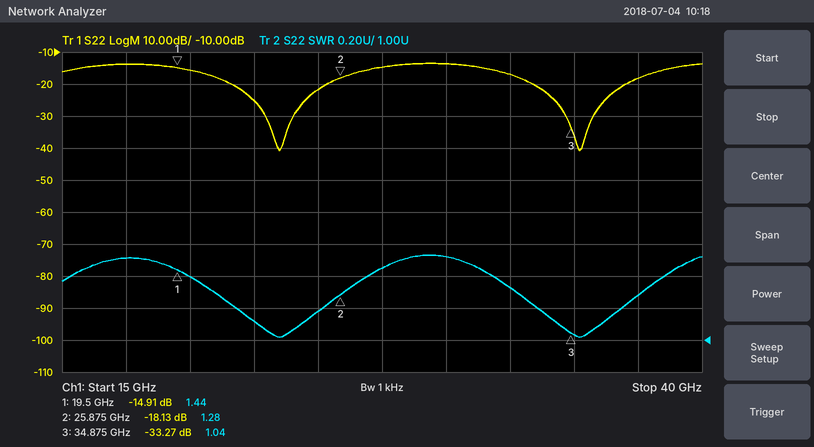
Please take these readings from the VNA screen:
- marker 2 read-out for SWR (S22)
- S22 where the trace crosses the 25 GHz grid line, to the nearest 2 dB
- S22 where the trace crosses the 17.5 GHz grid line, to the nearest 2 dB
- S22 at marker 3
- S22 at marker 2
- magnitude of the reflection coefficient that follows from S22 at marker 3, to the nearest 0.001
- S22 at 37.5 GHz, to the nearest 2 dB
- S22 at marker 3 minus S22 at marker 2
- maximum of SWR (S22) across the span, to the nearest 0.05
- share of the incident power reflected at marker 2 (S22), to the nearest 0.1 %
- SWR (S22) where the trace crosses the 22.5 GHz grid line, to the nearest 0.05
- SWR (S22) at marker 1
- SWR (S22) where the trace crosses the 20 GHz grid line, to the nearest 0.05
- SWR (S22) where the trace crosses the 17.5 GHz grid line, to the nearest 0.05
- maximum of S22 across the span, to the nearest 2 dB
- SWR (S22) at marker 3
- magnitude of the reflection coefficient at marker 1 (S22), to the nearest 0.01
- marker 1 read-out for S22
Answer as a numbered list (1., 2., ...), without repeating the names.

1. 1.28
2. -22 dB
3. -14 dB
4. -33.27 dB
5. -18.13 dB
6. 0.022
7. -18 dB
8. -15.14 dB
9. 1.55
10. 1.5 %
11. 1.10
12. 1.44
13. 1.40
14. 1.50
15. -14 dB
16. 1.04
17. 0.18
18. -14.91 dB
